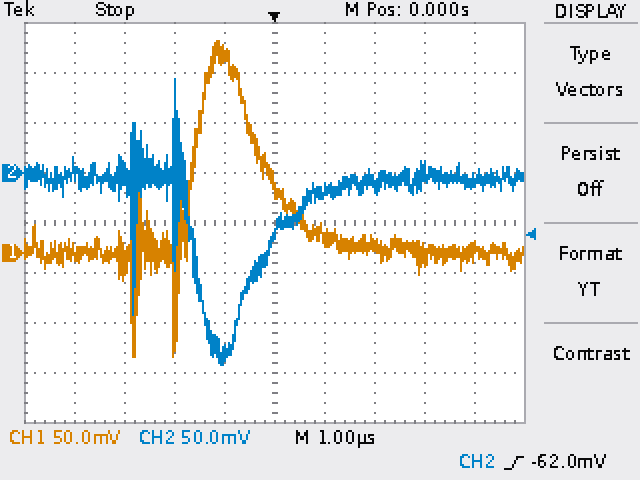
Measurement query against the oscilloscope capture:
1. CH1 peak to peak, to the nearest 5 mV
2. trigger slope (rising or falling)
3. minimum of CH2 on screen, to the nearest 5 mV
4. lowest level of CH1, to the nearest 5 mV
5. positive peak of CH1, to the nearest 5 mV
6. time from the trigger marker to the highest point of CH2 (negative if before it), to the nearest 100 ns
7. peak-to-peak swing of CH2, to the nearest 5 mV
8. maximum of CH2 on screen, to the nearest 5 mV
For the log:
315 mV
rising
-190 mV
-105 mV
210 mV
-2.0 µs
285 mV
95 mV
